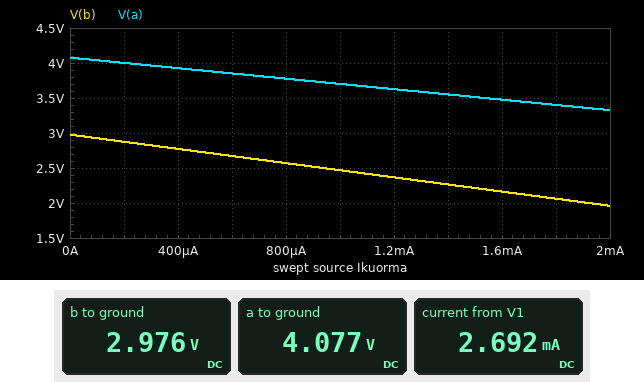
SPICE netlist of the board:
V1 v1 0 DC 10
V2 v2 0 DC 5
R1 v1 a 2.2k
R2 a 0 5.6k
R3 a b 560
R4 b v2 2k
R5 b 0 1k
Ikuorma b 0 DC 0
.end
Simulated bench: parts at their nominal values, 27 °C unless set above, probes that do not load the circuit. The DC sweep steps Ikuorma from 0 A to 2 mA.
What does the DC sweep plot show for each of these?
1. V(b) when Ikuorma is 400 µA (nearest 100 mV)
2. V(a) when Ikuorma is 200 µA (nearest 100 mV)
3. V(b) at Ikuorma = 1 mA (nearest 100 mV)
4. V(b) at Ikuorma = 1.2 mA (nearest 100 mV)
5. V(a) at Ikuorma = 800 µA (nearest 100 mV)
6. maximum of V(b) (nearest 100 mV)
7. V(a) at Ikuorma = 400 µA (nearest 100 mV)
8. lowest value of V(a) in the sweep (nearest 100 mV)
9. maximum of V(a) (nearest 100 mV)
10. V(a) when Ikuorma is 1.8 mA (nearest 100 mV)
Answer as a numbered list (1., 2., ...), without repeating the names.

1. 2.8 V
2. 4.0 V
3. 2.5 V
4. 2.4 V
5. 3.8 V
6. 3.0 V
7. 3.9 V
8. 3.3 V
9. 4.1 V
10. 3.4 V
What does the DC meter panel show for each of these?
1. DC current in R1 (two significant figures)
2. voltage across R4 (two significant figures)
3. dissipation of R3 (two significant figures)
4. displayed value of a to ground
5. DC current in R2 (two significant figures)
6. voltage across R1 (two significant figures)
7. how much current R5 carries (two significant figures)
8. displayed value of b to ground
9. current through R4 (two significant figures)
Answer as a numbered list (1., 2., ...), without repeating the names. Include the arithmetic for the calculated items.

1. (10 V - 4.077 V) / 2.2 kΩ = 2.7 mA
2. 5 V - 2.976 V = 2.0 V
3. (4.077 V - 2.976 V)^2 / 560 Ω = 2.2 mW
4. 4.077 V
5. (4.077 V) / 5.6 kΩ = 730 µA
6. 10 V - 4.077 V = 5.9 V
7. (2.976 V) / 1 kΩ = 3.0 mA
8. 2.976 V
9. (5 V - 2.976 V) / 2 kΩ = 1.0 mA
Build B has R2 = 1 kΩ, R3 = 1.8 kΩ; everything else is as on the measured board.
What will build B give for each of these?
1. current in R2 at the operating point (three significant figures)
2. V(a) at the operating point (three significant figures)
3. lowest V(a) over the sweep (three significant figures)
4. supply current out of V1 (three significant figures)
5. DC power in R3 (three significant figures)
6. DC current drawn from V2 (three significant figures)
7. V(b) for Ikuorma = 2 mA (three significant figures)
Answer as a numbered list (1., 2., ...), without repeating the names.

1. 2.81 mA
2. 2.81 V
3. 2.52 V
4. 3.27 mA
5. 385 µW
6. 1.51 mA
7. 923 mV
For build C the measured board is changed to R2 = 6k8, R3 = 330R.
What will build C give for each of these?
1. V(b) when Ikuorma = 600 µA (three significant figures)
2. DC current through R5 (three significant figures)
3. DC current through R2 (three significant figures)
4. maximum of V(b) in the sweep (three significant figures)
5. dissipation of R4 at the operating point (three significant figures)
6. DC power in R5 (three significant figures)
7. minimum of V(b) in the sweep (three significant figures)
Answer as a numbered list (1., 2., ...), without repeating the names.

1. 2.84 V
2. 3.14 mA
3. 570 µA
4. 3.14 V
5. 1.72 mW
6. 9.88 mW
7. 2.14 V
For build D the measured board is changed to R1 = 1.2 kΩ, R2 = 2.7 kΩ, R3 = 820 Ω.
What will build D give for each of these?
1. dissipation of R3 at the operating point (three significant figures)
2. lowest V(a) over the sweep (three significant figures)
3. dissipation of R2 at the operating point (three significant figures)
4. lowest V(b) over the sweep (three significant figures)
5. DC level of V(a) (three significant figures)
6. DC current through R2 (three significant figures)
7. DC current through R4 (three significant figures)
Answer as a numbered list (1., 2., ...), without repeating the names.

1. 4.22 mW
2. 4.56 V
3. 9.40 mW
4. 2.23 V
5. 5.04 V
6. 1.87 mA
7. 911 µA
